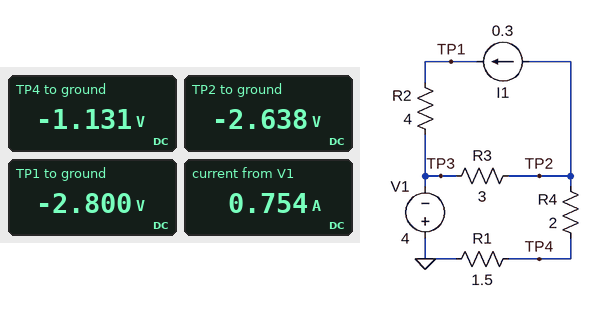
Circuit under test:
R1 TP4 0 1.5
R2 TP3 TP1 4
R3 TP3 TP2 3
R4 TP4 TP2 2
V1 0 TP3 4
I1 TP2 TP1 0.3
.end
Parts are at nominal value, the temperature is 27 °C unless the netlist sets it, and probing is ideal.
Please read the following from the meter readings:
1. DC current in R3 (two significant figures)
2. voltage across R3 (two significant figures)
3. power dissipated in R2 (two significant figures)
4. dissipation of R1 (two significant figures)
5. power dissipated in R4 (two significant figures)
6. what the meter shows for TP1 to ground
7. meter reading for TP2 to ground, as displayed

450 mA
1.4 V
360 mW
850 mW
1.1 W
-2.800 V
-2.638 V
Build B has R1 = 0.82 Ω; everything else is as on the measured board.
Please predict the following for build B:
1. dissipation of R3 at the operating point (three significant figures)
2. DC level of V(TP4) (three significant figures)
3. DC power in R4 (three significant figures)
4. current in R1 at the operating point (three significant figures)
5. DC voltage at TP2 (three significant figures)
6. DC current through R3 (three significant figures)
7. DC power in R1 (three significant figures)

881 mW
-690 mV
1.42 W
842 mA
-2.37 V
542 mA
581 mW
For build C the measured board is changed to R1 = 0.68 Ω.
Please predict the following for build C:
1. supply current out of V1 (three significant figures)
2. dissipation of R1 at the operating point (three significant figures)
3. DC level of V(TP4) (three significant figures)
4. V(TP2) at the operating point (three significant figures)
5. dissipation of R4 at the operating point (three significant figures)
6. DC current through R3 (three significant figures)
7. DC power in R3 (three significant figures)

863 mA
506 mW
-587 mV
-2.31 V
1.49 W
563 mA
950 mW
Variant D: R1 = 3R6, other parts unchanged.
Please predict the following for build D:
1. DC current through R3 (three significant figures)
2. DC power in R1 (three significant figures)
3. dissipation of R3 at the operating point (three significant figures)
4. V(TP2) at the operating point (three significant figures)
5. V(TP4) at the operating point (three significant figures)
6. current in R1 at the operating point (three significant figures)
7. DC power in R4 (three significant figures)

270 mA
1.17 W
218 mW
-3.19 V
-2.05 V
570 mA
649 mW
